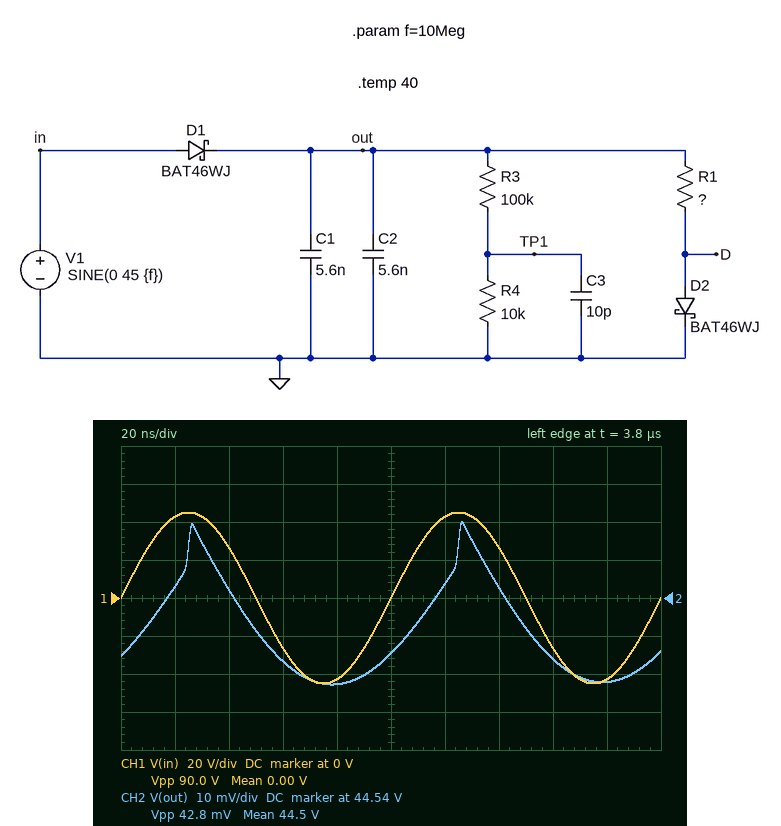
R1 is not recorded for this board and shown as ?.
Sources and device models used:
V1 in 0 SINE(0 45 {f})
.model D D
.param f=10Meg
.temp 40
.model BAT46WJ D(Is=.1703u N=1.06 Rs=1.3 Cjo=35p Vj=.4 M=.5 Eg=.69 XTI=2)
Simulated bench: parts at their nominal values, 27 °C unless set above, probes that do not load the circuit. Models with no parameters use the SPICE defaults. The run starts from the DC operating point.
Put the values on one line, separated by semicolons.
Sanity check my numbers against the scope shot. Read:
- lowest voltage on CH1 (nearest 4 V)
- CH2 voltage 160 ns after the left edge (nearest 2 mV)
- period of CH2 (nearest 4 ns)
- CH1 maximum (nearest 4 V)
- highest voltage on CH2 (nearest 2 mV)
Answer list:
-44 V; 44.524 V; 100 ns; 44 V; 44.560 V
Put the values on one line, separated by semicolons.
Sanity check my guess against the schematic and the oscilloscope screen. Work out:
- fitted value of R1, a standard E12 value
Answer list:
47 kΩ
